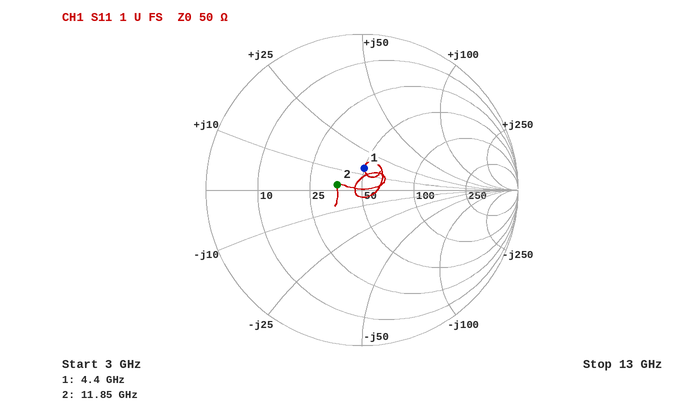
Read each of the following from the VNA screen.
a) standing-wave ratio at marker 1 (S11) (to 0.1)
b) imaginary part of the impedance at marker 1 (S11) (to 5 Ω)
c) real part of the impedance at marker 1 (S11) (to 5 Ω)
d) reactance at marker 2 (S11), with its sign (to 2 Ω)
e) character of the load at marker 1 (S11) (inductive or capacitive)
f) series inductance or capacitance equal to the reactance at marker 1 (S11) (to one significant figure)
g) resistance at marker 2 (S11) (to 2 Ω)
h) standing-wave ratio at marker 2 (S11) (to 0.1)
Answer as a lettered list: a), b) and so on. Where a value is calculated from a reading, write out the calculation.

a) 1.3
b) +15 Ω
c) 50 Ω
d) +2 Ω
e) inductive
f) L = 15 Ω/(2π × 4.4 GHz) ≈ 543 pH, so 500 pH to one significant figure
g) 36 Ω
h) 1.4
